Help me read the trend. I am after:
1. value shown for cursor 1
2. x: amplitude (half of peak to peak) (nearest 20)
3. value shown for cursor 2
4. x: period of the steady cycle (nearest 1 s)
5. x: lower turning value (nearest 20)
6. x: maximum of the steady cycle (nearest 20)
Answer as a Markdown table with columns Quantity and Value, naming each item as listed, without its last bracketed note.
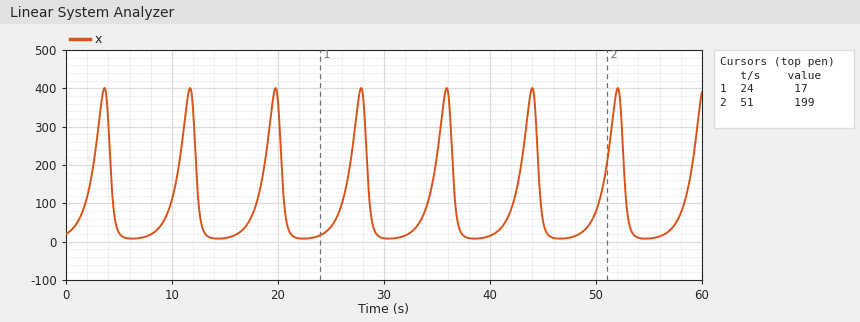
| Quantity | Value |
|---|---|
| value shown for cursor 1 | 17 |
| x: amplitude (half of peak to peak) | 200 |
| value shown for cursor 2 | 199 |
| x: period of the steady cycle | 8 s |
| x: lower turning value | 0 |
| x: maximum of the steady cycle | 400 |
